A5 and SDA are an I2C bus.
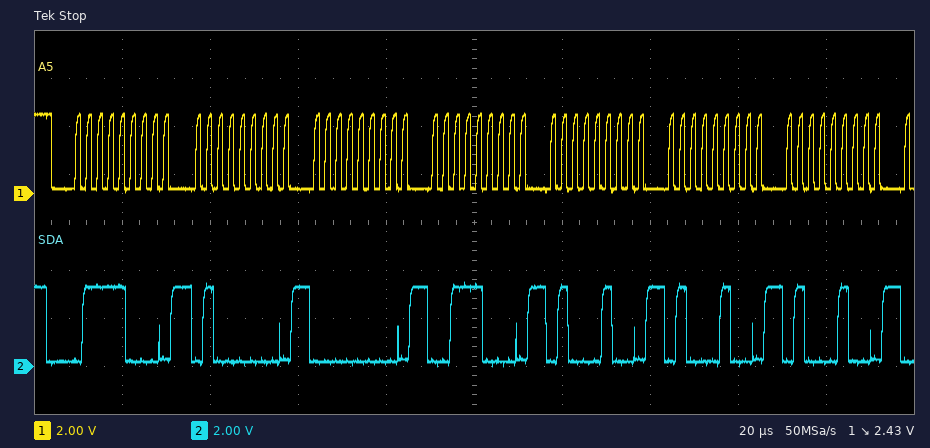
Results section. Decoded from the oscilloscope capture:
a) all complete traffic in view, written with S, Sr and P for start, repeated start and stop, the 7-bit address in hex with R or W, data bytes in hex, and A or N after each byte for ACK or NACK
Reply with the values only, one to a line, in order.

S 3CW A 40 A 00 A 38 A 44 A 44 A 44 A
